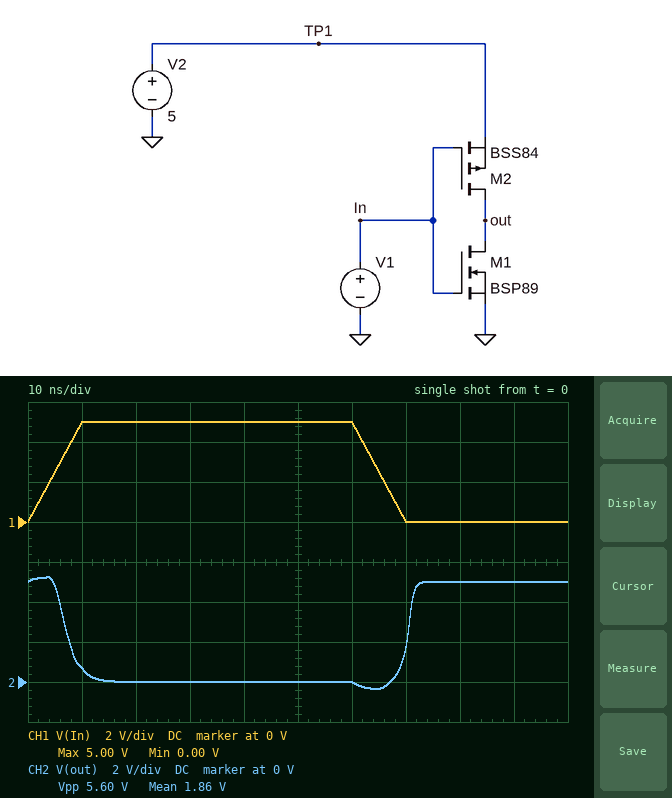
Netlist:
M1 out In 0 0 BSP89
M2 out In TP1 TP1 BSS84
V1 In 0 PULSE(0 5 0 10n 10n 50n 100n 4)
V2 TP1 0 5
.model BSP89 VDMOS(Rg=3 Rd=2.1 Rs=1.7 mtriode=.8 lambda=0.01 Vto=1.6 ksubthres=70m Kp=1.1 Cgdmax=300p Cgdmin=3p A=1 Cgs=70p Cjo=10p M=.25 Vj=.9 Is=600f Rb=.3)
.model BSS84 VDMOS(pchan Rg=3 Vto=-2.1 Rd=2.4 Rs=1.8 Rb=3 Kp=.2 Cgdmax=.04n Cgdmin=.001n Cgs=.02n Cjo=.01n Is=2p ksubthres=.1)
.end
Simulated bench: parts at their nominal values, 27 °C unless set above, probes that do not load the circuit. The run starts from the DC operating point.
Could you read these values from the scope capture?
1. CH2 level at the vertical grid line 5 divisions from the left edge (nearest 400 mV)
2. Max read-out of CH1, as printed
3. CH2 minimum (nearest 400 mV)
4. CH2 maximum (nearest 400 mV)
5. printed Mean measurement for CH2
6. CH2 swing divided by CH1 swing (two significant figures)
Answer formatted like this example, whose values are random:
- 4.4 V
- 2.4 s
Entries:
- 0 V
- 5.00 V
- -400 mV
- 5.2 V
- 1.86 V
- 1.1
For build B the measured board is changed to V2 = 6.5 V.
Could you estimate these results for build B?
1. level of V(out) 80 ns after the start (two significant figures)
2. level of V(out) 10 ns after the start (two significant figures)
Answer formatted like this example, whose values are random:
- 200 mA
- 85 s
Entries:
- 6.5 V
- 880 mV
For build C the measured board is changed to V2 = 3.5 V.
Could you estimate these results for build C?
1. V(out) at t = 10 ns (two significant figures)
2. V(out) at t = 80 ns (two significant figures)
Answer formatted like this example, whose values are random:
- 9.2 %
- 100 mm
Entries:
- 650 mV
- 3.5 V
